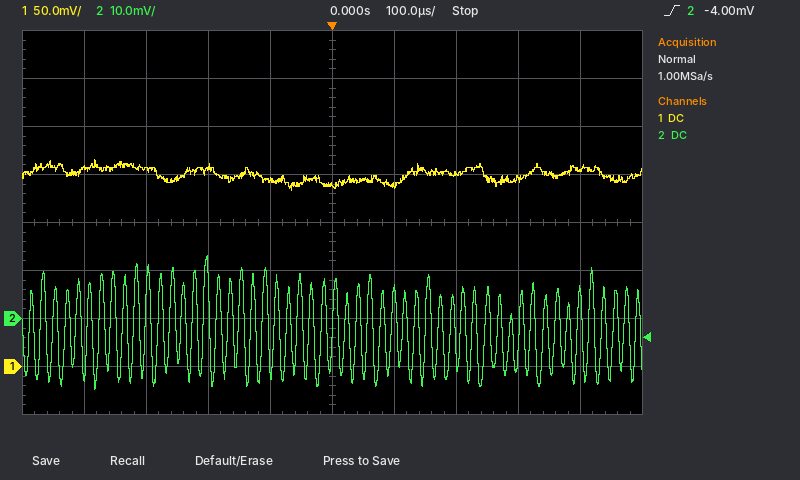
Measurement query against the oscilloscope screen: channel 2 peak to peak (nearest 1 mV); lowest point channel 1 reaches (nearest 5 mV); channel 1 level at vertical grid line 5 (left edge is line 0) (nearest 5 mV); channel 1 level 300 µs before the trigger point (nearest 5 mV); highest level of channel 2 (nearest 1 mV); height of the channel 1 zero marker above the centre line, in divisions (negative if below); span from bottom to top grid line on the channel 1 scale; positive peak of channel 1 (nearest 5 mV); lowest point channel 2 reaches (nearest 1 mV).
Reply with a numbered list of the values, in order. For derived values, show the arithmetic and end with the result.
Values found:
1. 13 mV − (-15 mV) = 28 mV
2. 185 mV
3. 190 mV
4. 205 mV
5. 13 mV
6. -3.0 div
7. 400 mV
8. 215 mV
9. -15 mV
